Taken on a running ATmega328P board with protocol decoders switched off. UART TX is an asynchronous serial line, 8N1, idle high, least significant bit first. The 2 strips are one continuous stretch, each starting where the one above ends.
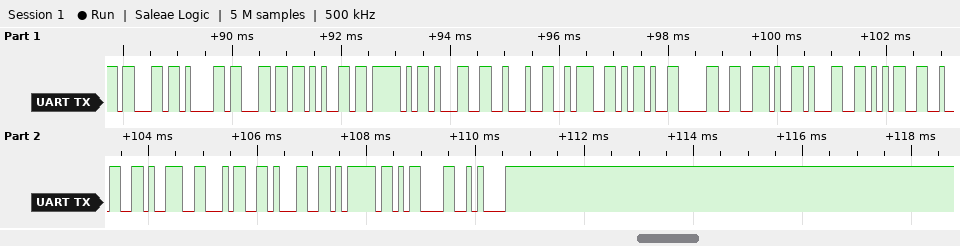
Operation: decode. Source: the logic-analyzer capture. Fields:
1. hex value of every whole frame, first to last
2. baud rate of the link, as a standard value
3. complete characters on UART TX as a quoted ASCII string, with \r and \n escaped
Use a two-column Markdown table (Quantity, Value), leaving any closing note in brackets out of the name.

| Quantity | Value |
|---|---|
| hex value of every whole frame, first to last | 63 61 6C 65 5F 31 22 3A 2D 30 2E 31 35 32 39 34 31 7D 0D 0A |
| baud rate of the link, as a standard value | 9600 baud |
| complete characters on UART TX as a quoted ASCII string, with \r and \n escaped | "cale_1\":-0.152941}\r\n" |
